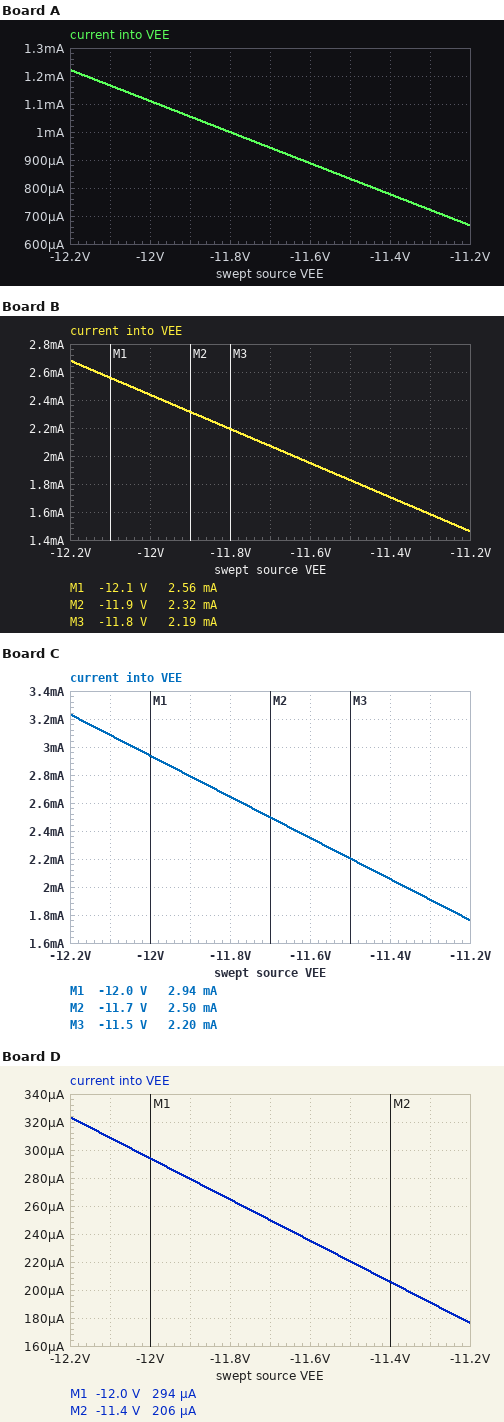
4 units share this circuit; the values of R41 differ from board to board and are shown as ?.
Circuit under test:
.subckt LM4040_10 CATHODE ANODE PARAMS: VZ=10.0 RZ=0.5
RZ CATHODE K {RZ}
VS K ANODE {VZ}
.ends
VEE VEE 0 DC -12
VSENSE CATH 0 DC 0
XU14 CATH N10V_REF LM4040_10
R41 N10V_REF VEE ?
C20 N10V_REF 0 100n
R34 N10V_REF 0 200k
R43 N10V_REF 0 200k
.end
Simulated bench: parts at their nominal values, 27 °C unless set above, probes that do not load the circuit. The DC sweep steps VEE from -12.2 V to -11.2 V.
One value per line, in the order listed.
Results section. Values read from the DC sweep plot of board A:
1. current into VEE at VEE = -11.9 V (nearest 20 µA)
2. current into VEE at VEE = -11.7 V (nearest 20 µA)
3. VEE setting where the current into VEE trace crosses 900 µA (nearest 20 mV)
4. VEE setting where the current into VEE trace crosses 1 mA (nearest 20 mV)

1.06 mA
940 µA
-11.62 V
-11.80 V
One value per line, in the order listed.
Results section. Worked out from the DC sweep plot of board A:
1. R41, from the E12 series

1.8 kΩ
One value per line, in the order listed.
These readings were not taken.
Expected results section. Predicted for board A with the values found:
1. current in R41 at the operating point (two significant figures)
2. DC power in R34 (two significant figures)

1.1 mA
500 µW
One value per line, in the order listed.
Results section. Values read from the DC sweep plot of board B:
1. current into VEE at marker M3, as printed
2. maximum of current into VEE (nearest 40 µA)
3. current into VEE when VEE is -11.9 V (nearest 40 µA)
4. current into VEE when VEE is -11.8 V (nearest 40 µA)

2.19 mA
2.68 mA
2.32 mA
2.20 mA
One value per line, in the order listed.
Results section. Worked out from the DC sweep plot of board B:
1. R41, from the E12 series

820 Ω
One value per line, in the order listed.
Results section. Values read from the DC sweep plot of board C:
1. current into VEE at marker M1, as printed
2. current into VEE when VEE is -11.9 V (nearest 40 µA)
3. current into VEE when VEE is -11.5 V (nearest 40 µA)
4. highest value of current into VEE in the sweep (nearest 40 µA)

2.94 mA
2.80 mA
2.20 mA
3.24 mA
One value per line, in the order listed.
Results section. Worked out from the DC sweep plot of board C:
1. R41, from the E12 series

680 Ω
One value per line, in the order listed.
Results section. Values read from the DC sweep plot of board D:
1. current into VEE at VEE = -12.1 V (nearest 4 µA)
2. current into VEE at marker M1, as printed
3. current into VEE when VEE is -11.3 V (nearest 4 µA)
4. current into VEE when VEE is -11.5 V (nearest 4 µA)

308 µA
294 µA
192 µA
220 µA
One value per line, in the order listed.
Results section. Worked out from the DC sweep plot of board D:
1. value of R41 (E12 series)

6.8 kΩ
